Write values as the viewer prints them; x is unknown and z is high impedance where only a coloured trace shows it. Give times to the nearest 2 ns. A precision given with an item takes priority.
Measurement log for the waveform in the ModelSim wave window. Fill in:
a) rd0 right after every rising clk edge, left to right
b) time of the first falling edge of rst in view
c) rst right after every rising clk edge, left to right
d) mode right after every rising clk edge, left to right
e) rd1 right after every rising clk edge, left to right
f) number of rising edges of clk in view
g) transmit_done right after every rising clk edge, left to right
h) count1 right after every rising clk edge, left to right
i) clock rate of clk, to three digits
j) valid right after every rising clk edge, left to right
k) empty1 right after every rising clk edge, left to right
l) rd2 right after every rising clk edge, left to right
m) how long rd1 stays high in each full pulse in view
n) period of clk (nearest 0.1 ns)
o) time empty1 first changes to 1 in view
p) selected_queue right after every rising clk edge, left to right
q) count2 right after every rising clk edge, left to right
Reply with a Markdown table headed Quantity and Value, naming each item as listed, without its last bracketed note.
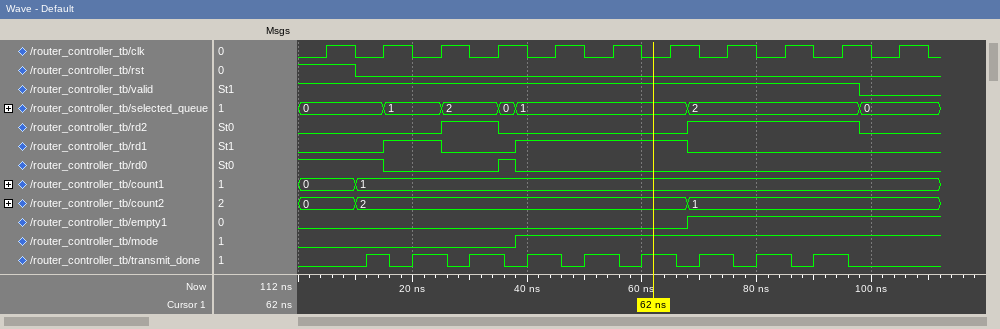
| Quantity | Value |
|---|---|
| rd0 right after every rising clk edge, left to right | 1 0 0 1 0 0 0 0 0 0 0 |
| time of the first falling edge of rst in view | 10 ns |
| rst right after every rising clk edge, left to right | 1 0 0 0 0 0 0 0 0 0 0 |
| mode right after every rising clk edge, left to right | 0 0 0 0 1 1 1 1 1 1 1 |
| rd1 right after every rising clk edge, left to right | 0 1 0 0 1 1 1 0 0 0 0 |
| number of rising edges of clk in view | 11 |
| transmit_done right after every rising clk edge, left to right | 0 1 1 1 1 1 1 1 1 1 0 |
| count1 right after every rising clk edge, left to right | 0, 1, 1, 1, 1, 1, 1, 1, 1, 1, 1 |
| clock rate of clk, to three digits | 100 MHz |
| valid right after every rising clk edge, left to right | 1 1 1 1 1 1 1 1 1 1 0 |
| empty1 right after every rising clk edge, left to right | 0 0 0 0 0 0 0 1 1 1 1 |
| rd2 right after every rising clk edge, left to right | 0 0 1 0 0 0 0 1 1 1 0 |
| how long rd1 stays high in each full pulse in view | 10 ns, 30 ns |
| period of clk | 10 ns |
| time empty1 first changes to 1 in view | 68 ns |
| selected_queue right after every rising clk edge, left to right | 0, 1, 2, 0, 1, 1, 1, 2, 2, 2, 0 |
| count2 right after every rising clk edge, left to right | 0, 2, 2, 2, 2, 2, 2, 1, 1, 1, 1 |
